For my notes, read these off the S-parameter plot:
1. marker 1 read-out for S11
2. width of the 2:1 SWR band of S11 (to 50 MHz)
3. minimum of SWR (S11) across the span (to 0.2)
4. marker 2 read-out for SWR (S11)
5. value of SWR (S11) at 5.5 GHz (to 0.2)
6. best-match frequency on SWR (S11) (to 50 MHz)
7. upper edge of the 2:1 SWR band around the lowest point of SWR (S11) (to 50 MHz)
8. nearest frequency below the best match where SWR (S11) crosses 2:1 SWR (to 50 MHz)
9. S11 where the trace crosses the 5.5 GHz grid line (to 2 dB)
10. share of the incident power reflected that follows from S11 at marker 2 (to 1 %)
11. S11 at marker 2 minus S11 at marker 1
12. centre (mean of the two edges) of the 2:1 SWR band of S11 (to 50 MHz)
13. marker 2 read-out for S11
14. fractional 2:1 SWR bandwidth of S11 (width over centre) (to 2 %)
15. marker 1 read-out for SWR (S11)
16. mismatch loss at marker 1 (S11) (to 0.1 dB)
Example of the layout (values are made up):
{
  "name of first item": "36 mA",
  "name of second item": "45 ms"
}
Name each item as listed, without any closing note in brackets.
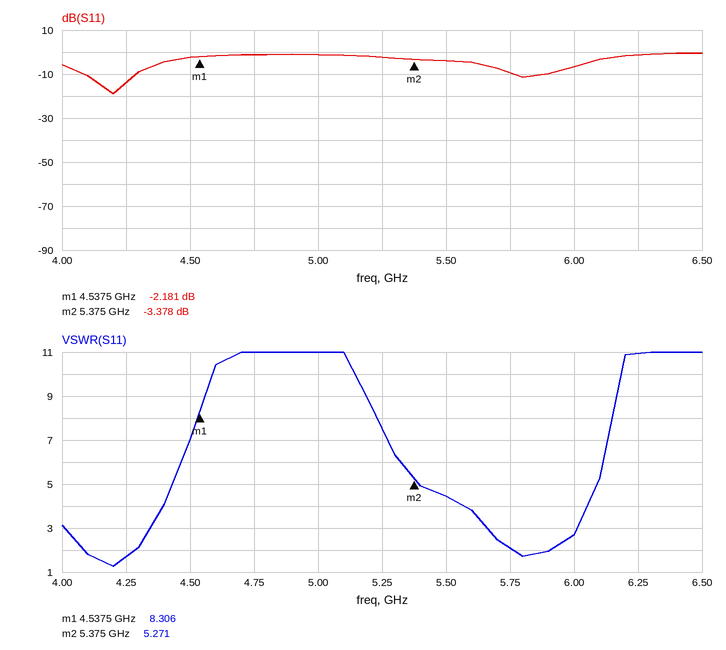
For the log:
{
  "marker 1 read-out for S11": "-2.181 dB",
  "width of the 2:1 SWR band of S11": "200 MHz",
  "minimum of SWR (S11) across the span": "1.2",
  "marker 2 read-out for SWR": "5.271",
  "value of SWR (S11) at 5.5 GHz": "4.4",
  "best-match frequency on SWR (S11)": "4.20 GHz",
  "upper edge of the 2:1 SWR band around the lowest point of SWR (S11)": "4.30 GHz",
  "nearest frequency below the best match where SWR (S11) crosses 2:1 SWR": "4.10 GHz",
  "S11 where the trace crosses the 5.5 GHz grid line": "-4 dB",
  "share of the incident power reflected that follows from S11 at marker 2": "46 %",
  "S11 at marker 2 minus S11 at marker 1": "-1.197 dB",
  "centre (mean of the two edges) of the 2:1 SWR band of S11": "4.20 GHz",
  "marker 2 read-out for S11": "-3.378 dB",
  "fractional 2:1 SWR bandwidth of S11 (width over centre)": "4 %",
  "marker 1 read-out for SWR": "8.306",
  "mismatch loss at marker 1 (S11)": "4.0 dB"
}
